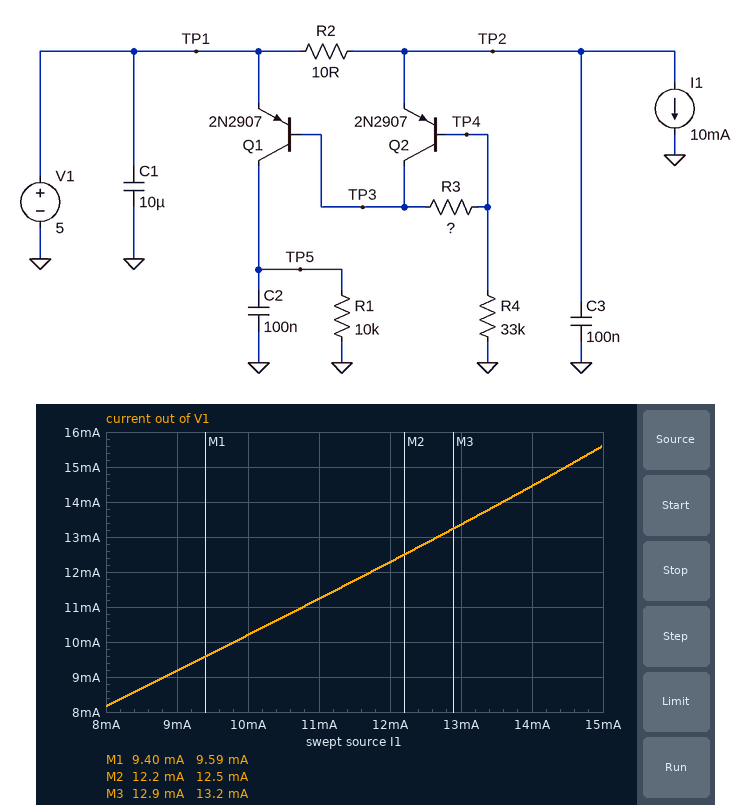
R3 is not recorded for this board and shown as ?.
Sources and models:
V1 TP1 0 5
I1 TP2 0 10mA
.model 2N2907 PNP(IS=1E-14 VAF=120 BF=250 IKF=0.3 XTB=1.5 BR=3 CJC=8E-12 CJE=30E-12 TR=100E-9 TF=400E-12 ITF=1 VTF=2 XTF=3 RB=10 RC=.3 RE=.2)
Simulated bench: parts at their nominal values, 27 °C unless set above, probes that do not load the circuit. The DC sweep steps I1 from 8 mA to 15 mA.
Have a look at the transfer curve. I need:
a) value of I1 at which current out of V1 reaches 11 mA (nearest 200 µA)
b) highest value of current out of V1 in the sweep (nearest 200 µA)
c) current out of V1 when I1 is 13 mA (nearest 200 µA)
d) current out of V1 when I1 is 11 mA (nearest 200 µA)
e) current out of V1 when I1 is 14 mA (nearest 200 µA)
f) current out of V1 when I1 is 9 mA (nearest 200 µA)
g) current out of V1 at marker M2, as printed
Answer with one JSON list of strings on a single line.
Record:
["10.8 mA", "15.6 mA", "13.4 mA", "11.2 mA", "14.4 mA", "9.2 mA", "12.5 mA"]
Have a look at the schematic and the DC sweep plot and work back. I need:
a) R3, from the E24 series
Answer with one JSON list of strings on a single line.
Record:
["910 Ω"]
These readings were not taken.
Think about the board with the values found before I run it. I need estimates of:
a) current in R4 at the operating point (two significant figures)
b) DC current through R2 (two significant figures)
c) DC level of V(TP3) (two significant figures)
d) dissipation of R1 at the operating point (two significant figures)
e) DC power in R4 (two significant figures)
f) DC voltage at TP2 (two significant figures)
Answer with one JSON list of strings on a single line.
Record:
["130 µA", "10 mA", "4.4 V", "49 µW", "560 µW", "4.9 V"]
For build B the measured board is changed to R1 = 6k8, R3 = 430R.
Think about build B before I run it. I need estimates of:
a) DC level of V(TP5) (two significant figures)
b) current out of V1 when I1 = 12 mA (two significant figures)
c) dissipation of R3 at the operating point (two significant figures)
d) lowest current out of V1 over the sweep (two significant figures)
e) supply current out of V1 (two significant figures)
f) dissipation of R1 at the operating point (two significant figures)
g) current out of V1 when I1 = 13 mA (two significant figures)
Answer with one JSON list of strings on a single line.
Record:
["4.9 V", "13 mA", "7.2 µW", "8.5 mA", "11 mA", "3.5 mW", "14 mA"]
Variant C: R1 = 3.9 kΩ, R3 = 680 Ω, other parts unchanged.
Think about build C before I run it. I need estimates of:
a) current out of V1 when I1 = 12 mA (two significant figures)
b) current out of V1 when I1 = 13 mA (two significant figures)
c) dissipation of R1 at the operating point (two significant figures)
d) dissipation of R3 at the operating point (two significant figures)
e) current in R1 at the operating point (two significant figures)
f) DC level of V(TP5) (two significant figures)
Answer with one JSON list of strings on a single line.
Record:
["13 mA", "14 mA", "190 µW", "11 µW", "220 µA", "860 mV"]
